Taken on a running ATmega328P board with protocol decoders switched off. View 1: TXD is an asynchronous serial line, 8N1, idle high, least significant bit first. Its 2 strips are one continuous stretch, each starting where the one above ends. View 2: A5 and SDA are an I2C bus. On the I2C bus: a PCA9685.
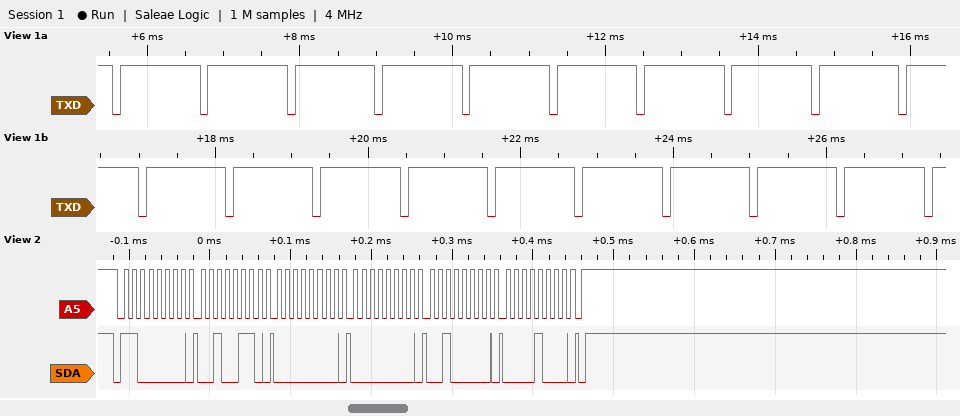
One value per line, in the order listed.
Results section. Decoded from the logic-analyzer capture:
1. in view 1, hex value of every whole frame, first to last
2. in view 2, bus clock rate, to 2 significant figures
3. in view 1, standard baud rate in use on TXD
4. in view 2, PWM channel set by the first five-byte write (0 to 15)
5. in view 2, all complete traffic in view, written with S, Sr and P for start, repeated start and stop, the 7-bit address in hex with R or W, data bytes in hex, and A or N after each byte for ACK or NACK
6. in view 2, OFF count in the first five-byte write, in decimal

FF FF FF FF FF FF FF FF FF FF FF FF FF FF FF FF FF FF FF
100 kHz
9600 baud
8
S 60W A 26 A 00 A 00 A 20 A 08 A P
2080
